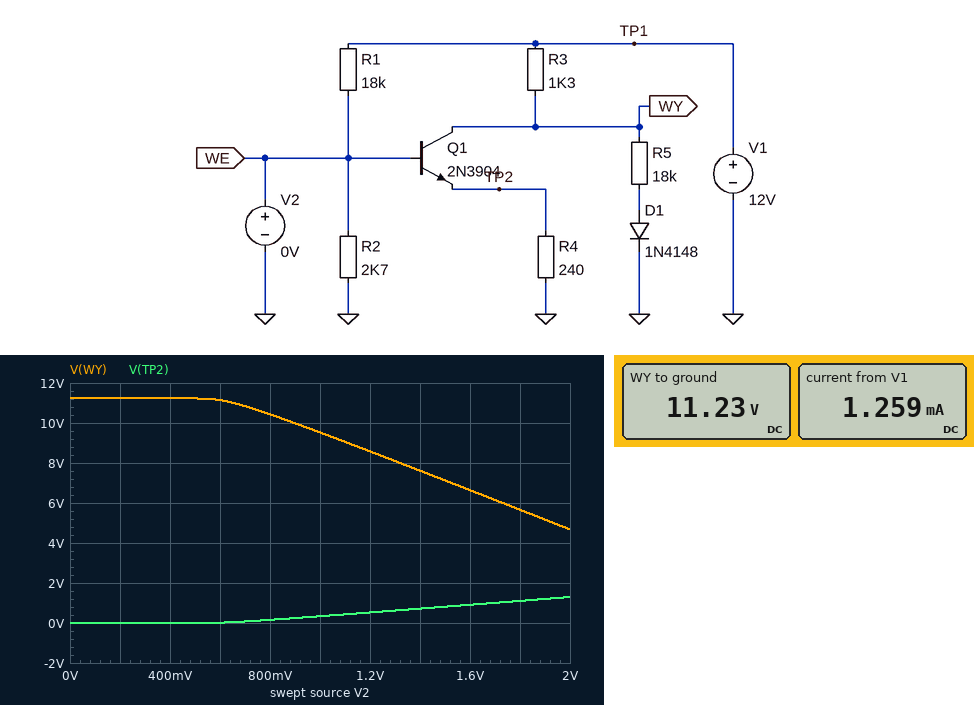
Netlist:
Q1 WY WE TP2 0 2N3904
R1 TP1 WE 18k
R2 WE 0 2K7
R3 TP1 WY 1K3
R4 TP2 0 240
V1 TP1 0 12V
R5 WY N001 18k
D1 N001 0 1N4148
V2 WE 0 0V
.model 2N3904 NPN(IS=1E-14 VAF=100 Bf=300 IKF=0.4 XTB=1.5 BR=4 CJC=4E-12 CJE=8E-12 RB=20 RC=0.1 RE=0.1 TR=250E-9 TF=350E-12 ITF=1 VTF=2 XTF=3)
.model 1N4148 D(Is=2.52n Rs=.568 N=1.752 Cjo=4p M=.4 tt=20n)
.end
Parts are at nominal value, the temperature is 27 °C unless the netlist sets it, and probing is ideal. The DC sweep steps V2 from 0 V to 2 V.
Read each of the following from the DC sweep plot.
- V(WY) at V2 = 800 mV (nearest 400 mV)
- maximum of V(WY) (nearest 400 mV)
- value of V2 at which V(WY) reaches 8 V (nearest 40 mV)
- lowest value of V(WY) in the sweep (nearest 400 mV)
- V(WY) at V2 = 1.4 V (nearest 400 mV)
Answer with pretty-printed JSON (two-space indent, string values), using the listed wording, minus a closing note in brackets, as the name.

{
  "V(WY) at V2 = 800 mV": "10.4 V",
  "maximum of V(WY)": "11.2 V",
  "value of V2 at which V(WY) reaches 8 V": "1.32 V",
  "lowest value of V(WY) in the sweep": "4.8 V",
  "V(WY) at V2 = 1.4 V": "7.6 V"
}
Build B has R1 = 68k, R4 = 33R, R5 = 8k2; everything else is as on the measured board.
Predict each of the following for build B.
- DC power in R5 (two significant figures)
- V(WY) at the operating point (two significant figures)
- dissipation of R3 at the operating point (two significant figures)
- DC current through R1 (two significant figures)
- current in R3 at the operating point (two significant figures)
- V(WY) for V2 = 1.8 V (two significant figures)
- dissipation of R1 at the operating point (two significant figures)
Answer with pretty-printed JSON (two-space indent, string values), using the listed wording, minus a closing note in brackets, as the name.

{
  "DC power in R5": "12 mW",
  "V(WY) at the operating point": "10 V",
  "dissipation of R3 at the operating point": "1.9 mW",
  "DC current through R1": "180 µA",
  "current in R3 at the operating point": "1.2 mA",
  "V(WY) for V2 = 1.8 V": "760 mV",
  "dissipation of R1 at the operating point": "2.1 mW"
}
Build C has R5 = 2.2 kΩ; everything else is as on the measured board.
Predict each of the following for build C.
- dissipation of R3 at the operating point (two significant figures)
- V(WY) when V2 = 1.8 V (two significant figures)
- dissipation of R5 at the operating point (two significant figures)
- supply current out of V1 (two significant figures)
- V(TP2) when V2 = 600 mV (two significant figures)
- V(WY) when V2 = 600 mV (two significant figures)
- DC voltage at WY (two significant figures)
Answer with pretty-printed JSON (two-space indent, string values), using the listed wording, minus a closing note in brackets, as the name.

{
  "dissipation of R3 at the operating point": "14 mW",
  "V(WY) when V2 = 1.8 V": "4.0 V",
  "dissipation of R5 at the operating point": "23 mW",
  "supply current out of V1": "3.9 mA",
  "V(TP2) when V2 = 600 mV": "16 mV",
  "V(WY) when V2 = 600 mV": "7.7 V",
  "DC voltage at WY": "7.8 V"
}
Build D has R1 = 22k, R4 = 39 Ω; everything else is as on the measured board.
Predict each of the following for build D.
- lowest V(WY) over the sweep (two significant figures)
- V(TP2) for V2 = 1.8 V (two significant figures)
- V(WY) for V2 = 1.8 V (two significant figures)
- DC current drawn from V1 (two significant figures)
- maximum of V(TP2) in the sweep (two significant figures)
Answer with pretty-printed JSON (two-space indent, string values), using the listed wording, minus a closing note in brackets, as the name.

{
  "lowest V(WY) over the sweep": "420 mV",
  "V(TP2) for V2 = 1.8 V": "800 mV",
  "V(WY) for V2 = 1.8 V": "810 mV",
  "DC current drawn from V1": "1.1 mA",
  "maximum of V(TP2) in the sweep": "920 mV"
}
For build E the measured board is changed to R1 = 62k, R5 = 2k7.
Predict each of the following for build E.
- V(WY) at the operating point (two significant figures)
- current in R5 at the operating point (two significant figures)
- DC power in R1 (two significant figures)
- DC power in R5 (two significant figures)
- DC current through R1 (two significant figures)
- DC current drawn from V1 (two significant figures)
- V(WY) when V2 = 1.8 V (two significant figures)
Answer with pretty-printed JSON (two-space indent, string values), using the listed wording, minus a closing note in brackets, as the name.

{
  "V(WY) at the operating point": "8.3 V",
  "current in R5 at the operating point": "2.8 mA",
  "DC power in R1": "2.3 mW",
  "DC power in R5": "22 mW",
  "DC current through R1": "190 µA",
  "DC current drawn from V1": "3.0 mA",
  "V(WY) when V2 = 1.8 V": "4.3 V"
}
